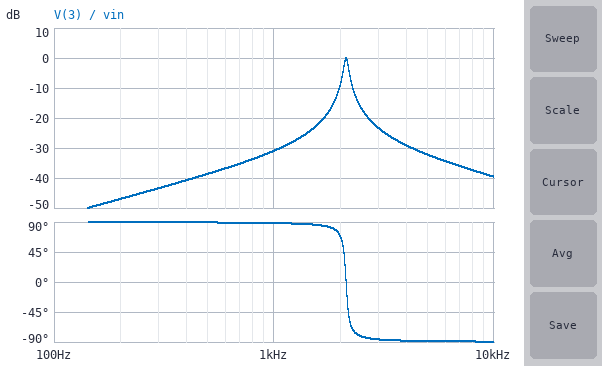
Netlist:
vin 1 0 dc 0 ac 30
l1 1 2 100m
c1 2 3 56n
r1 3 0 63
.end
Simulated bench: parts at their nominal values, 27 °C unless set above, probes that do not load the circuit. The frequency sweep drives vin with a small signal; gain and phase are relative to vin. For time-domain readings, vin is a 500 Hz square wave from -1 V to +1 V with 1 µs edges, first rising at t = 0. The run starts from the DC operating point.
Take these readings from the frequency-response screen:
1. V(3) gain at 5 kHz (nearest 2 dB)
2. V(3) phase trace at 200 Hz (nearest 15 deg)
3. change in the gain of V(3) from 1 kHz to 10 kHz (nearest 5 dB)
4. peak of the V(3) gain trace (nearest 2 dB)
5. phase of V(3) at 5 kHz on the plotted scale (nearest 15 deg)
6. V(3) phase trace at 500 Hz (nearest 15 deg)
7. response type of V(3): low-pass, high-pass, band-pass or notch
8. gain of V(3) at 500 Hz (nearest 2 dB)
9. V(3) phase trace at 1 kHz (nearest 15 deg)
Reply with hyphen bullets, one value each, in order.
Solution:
- -32 dB
- 90 deg
- -10 dB
- 0 dB
- -90 deg
- 90 deg
- band-pass
- -38 dB
- 90 deg
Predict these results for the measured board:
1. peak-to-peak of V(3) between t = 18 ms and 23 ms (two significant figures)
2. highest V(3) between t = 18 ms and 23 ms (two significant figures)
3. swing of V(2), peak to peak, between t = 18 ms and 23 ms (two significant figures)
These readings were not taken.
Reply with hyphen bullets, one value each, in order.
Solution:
- 110 mV
- 56 mV
- 4.3 V
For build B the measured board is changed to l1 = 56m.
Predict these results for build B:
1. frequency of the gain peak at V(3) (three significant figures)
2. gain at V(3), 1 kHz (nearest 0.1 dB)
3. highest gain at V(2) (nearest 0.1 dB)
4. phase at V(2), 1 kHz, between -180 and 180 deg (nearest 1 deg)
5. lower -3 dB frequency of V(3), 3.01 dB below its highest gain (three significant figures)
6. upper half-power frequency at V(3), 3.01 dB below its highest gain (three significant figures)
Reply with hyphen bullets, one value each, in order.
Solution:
- 2.84 kHz
- -31.9 dB
- 24.0 dB
- 0 deg
- 2.75 kHz
- 2.93 kHz
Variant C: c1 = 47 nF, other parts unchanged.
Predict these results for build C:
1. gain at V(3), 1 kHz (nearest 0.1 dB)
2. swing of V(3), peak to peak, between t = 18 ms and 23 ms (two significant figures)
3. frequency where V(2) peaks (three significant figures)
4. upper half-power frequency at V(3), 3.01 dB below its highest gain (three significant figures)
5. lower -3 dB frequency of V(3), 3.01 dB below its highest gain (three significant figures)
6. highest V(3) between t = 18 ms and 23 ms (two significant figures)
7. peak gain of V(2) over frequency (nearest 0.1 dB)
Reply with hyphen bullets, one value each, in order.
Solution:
- -32.8 dB
- 170 mV
- 2.32 kHz
- 2.37 kHz
- 2.27 kHz
- 86 mV
- 27.3 dB
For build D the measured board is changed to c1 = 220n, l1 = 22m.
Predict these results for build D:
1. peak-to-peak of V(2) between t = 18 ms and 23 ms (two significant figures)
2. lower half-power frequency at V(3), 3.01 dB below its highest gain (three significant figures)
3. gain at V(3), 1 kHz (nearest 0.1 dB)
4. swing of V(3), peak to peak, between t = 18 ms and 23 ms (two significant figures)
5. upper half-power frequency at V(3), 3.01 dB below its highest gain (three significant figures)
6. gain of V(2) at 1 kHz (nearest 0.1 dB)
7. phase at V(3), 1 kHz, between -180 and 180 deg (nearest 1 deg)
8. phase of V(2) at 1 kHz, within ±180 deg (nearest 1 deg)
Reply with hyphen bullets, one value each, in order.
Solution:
- 4.9 V
- 2.07 kHz
- -19.4 dB
- 680 mV
- 2.53 kHz
- 1.8 dB
- 84 deg
- -1 deg
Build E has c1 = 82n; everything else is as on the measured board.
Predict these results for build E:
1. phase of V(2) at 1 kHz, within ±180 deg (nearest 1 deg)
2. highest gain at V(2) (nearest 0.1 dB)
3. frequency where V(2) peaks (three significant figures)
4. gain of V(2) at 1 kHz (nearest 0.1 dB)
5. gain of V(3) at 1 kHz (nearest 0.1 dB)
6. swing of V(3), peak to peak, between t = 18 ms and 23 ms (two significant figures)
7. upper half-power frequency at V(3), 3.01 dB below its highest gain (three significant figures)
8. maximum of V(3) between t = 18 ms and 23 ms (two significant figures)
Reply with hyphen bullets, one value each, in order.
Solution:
- -1 deg
- 24.9 dB
- 1.76 kHz
- 3.4 dB
- -26.4 dB
- 180 mV
- 1.81 kHz
- 88 mV
